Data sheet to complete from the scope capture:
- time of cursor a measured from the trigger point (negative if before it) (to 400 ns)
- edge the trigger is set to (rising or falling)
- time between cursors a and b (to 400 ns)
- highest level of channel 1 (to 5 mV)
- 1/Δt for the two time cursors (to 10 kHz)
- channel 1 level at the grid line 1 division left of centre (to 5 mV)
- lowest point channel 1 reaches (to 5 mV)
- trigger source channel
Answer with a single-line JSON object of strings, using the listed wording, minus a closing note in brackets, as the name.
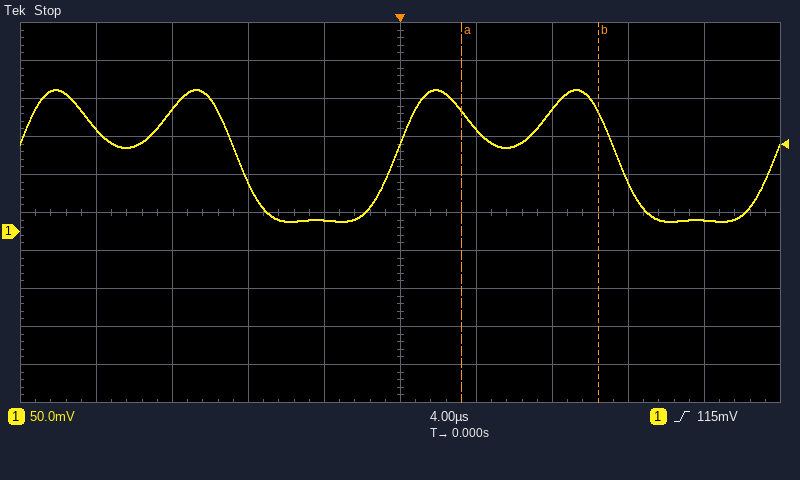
{"time of cursor a measured from the trigger point (negative if before it)": "+3.2 µs", "edge the trigger is set to": "rising", "time between cursors a and b": "7.2 µs", "highest level of channel 1": "185 mV", "1/Δt for the two time cursors": "140 kHz", "channel 1 level at the grid line 1 division left of centre": "15 mV", "lowest point channel 1 reaches": "15 mV", "trigger source channel": "channel 1"}
